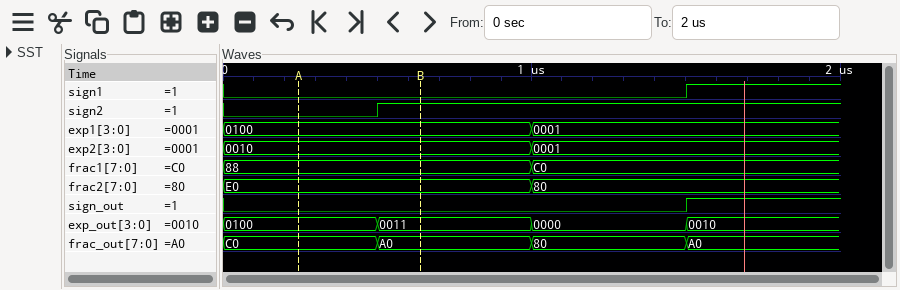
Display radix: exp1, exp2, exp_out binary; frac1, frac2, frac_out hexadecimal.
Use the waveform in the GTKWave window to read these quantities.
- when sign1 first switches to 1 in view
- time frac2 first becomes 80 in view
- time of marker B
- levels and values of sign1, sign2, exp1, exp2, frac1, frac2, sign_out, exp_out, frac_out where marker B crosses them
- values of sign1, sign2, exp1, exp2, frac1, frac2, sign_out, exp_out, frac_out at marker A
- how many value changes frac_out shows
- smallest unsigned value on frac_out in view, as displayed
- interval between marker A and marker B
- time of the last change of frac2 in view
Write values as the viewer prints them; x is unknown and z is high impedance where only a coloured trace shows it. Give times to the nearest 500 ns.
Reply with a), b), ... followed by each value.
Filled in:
a) 1500 ns
b) 1000 ns
c) 500 ns
d) sign1=0, sign2=1, exp1=0100, exp2=0010, frac1=88, frac2=E0, sign_out=0, exp_out=0011, frac_out=A0
e) sign1=0, sign2=0, exp1=0100, exp2=0010, frac1=88, frac2=E0, sign_out=0, exp_out=0100, frac_out=C0
f) 3
g) 80
h) 500 ns
i) 1000 ns
